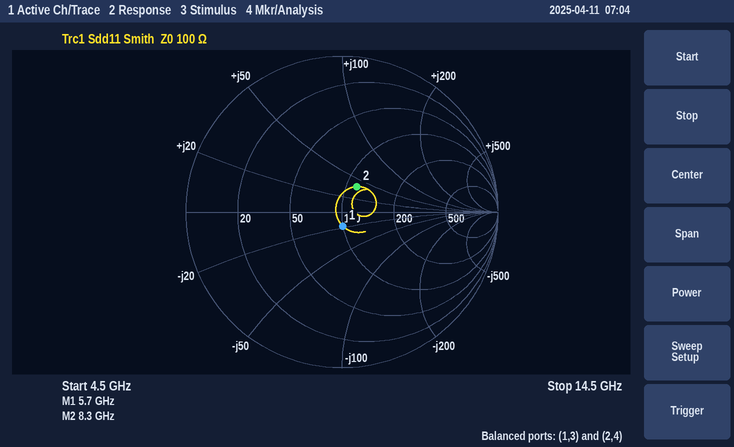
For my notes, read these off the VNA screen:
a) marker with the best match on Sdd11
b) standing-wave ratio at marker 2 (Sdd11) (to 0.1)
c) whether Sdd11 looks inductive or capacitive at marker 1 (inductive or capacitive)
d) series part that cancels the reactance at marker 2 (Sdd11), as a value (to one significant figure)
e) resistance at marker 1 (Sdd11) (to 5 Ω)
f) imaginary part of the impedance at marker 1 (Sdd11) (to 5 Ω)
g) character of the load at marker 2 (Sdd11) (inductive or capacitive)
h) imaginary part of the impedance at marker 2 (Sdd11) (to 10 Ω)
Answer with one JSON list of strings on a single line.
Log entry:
["marker 1", "1.5", "capacitive", "500 fF", "100 Ω", "-20 Ω", "inductive", "+40 Ω"]
